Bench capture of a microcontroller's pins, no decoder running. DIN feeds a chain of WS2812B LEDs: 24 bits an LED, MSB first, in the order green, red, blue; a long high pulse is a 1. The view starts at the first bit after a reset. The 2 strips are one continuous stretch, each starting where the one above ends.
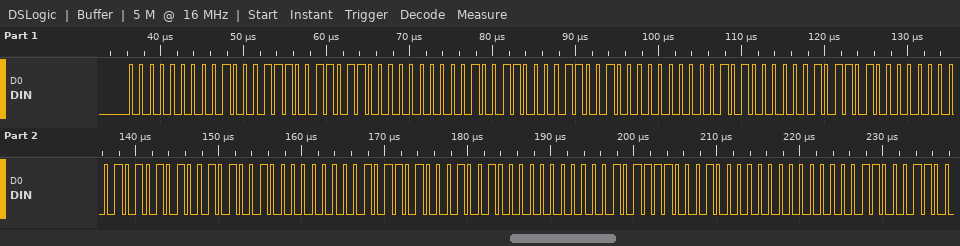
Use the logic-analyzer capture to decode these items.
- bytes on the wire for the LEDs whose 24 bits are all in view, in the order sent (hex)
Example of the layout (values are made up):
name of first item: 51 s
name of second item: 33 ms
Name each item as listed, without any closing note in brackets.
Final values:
bytes on the wire for the LEDs whose 24 bits are all in view, in the order sent: 00 47 36 00 4C 32 00 50 2D 00 55 29 00 5A 24 00 5E 20
